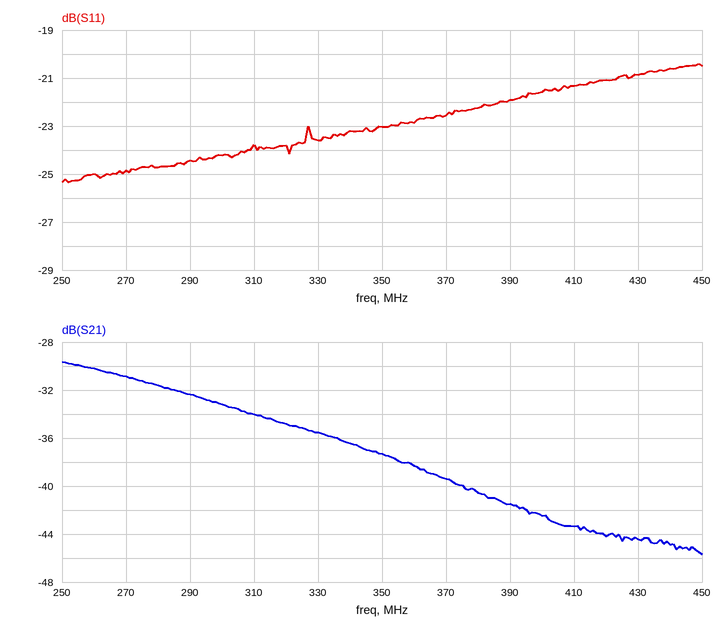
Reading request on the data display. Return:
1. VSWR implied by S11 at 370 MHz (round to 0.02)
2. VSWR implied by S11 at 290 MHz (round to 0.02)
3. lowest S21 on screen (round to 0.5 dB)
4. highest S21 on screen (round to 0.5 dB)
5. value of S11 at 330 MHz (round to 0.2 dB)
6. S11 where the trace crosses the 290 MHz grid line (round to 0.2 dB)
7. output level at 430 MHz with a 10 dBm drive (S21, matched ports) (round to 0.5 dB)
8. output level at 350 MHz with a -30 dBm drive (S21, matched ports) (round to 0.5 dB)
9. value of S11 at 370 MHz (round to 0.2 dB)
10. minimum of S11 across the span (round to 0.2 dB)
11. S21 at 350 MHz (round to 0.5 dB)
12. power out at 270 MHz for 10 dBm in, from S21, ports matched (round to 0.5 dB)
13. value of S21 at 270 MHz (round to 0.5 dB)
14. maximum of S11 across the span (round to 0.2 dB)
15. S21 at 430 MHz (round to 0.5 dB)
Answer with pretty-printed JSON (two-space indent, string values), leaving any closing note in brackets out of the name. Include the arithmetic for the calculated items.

{
  "VSWR implied by S11 at 370 MHz": "|Γ| = 10^(-22.6/20) = 0.0741; VSWR = (1 + 0.0741)/(1 − 0.0741) ≈ 1.16",
  "VSWR implied by S11 at 290 MHz": "|Γ| = 10^(-24.4/20) = 0.0603; VSWR = (1 + 0.0603)/(1 − 0.0603) ≈ 1.13, so 1.12 to the nearest 0.02",
  "lowest S21 on screen": "-45.5 dB",
  "highest S21 on screen": "-29.5 dB",
  "value of S11 at 330 MHz": "-23.6 dB",
  "S11 where the trace crosses the 290 MHz grid line": "-24.4 dB",
  "output level at 430 MHz with a 10 dBm drive (S21, matched ports)": "10 dBm + (-44.5 dB) = -34.5 dBm",
  "output level at 350 MHz with a -30 dBm drive (S21, matched ports)": "-30 dBm + (-37.5 dB) = -67.5 dBm",
  "value of S11 at 370 MHz": "-22.6 dB",
  "minimum of S11 across the span": "-25.4 dB",
  "S21 at 350 MHz": "-37.5 dB",
  "power out at 270 MHz for 10 dBm in, from S21, ports matched": "10 dBm + (-31.0 dB) = -21.0 dBm",
  "value of S21 at 270 MHz": "-31.0 dB",
  "maximum of S11 across the span": "-20.4 dB",
  "S21 at 430 MHz": "-44.5 dB"
}
